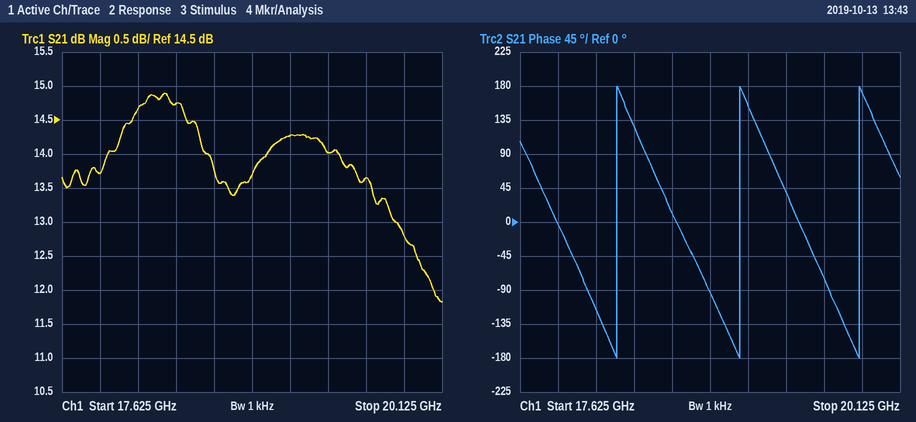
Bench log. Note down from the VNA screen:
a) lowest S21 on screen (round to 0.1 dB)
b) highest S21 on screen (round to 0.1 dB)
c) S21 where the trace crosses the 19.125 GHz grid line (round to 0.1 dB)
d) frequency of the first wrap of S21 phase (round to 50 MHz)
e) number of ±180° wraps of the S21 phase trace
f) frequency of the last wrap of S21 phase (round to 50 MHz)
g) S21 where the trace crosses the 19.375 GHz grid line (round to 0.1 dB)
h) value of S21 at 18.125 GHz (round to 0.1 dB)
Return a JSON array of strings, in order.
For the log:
["11.8 dB", "14.9 dB", "14.3 dB", "18.25 GHz", "3", "19.85 GHz", "14.0 dB", "14.7 dB"]
